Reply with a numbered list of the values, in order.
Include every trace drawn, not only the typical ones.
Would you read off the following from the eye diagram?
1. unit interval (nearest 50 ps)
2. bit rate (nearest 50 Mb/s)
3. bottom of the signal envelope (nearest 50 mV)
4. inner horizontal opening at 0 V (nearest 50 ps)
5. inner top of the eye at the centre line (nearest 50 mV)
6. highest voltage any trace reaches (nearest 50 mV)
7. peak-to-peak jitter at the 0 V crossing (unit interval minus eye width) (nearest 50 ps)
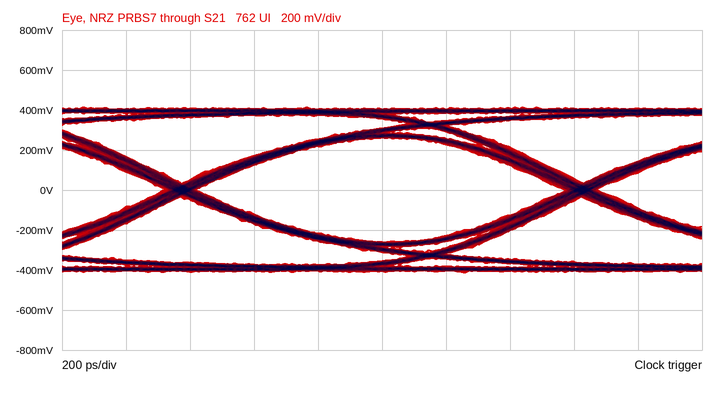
1. 1.25 ns
2. 800 Mb/s
3. -400 mV
4. 1.15 ns
5. 250 mV
6. 400 mV
7. 100 ps
